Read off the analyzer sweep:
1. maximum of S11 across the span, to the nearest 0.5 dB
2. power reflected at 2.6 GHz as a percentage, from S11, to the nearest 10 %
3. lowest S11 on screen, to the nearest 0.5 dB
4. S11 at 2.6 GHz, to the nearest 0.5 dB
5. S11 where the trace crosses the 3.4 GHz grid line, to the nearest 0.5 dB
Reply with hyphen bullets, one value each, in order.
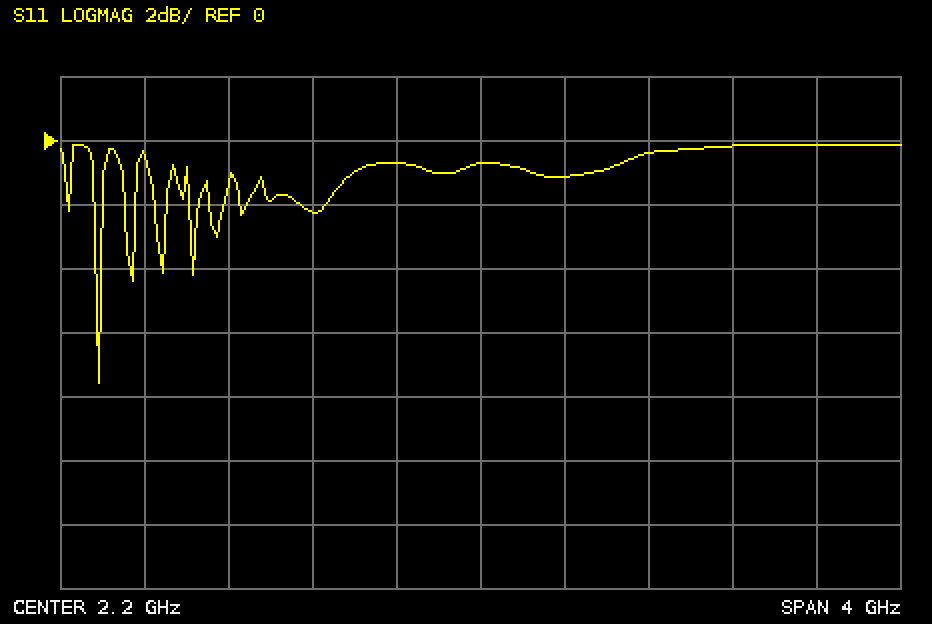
- 0.0 dB
- 80 %
- -7.5 dB
- -1.0 dB
- 0.0 dB
